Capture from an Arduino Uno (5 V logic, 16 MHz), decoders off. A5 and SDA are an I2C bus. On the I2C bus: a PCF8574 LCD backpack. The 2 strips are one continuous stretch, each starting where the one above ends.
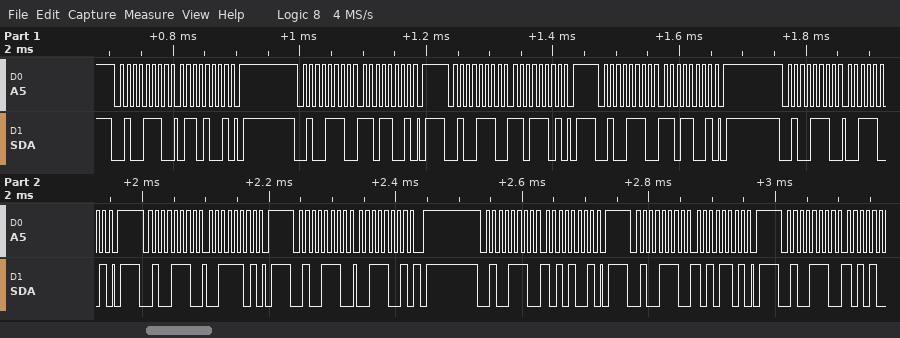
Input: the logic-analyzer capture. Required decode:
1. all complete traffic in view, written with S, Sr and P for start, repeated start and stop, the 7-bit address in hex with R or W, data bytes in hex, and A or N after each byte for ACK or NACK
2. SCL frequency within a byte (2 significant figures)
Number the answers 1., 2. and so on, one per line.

1. S 27W A 69 A P S 27W A D9 A P S 27W A DD A P S 27W A D9 A P S 27W A 39 A P S 27W A 3D A P S 27W A 39 A P S 27W A A9 A P S 27W A AD A P S 27W A
2. 100 kHz
